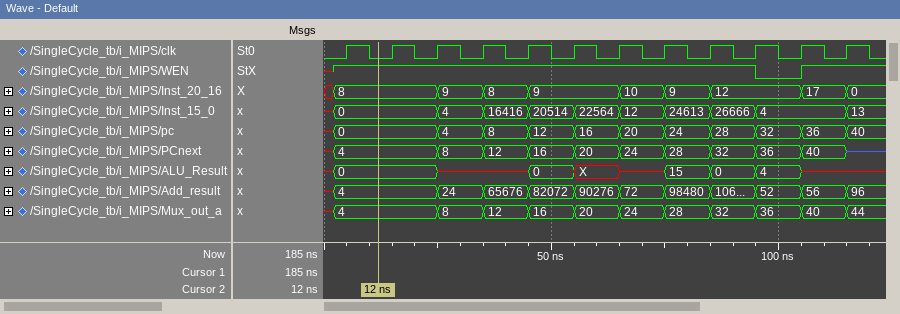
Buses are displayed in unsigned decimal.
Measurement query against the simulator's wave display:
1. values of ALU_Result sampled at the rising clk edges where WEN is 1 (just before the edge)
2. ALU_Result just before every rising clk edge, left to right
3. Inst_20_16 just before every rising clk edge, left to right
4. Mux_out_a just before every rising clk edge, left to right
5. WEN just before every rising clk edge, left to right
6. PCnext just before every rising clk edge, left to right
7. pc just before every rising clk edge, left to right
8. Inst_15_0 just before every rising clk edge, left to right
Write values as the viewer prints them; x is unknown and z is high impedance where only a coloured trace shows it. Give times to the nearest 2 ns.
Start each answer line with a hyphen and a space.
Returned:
- 0, 0, 0, x, x, 0, X, x, 15, 0, x
- 0, 0, 0, x, x, 0, X, x, 15, 0, 4, x
- 8, 8, 8, 9, 8, 9, 9, 10, 9, 12, 12, 17
- 4, 4, 4, 8, 12, 16, 20, 24, 28, 32, 36, 40
- 1 1 1 1 1 1 1 1 1 1 0 1
- 4, 4, 4, 8, 12, 16, 20, 24, 28, 32, 36, 40
- 0, 0, 0, 4, 8, 12, 16, 20, 24, 28, 32, 36
- 0, 0, 0, 4, 16416, 20514, 22564, 12, 24613, 26666, 4, 4
